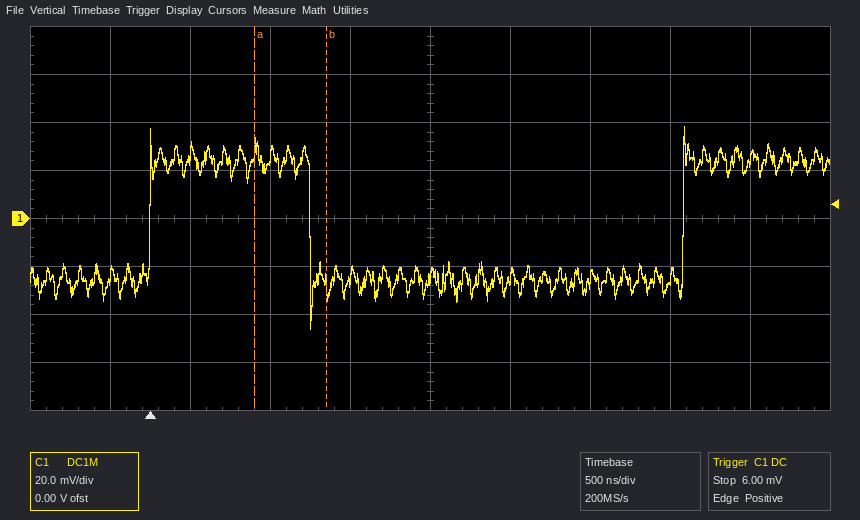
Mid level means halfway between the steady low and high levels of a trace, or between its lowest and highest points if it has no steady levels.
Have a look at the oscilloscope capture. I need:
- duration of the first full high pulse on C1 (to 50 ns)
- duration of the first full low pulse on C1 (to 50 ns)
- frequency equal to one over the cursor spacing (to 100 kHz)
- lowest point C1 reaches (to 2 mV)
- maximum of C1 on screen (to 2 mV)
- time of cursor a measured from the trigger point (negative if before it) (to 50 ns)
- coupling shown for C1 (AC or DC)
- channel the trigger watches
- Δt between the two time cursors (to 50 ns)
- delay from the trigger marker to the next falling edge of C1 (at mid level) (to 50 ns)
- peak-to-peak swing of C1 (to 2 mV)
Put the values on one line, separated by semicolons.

1.00 µs; 2.35 µs; 2.2 MHz; -46 mV; 38 mV; +650 ns; DC; C1; 450 ns; 1.00 µs; 84 mV
